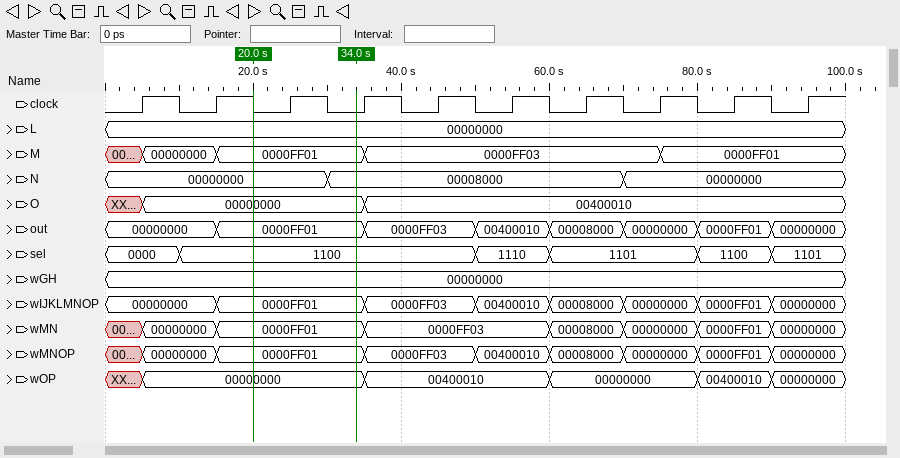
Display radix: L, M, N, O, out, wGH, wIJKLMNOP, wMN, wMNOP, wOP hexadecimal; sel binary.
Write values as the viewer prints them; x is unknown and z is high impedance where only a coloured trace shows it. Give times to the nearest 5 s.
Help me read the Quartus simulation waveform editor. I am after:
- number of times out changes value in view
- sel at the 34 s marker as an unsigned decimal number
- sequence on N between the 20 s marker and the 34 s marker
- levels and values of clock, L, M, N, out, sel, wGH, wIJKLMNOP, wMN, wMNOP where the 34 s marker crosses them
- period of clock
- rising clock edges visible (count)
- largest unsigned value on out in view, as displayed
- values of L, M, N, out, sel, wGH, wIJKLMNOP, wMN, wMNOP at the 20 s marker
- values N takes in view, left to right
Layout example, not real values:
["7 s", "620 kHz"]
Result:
["7", "12", "00000000, 00008000", "clock=0, L=00000000, M=0000FF01, N=00008000, out=0000FF01, sel=1100, wGH=00000000, wIJKLMNOP=0000FF01, wMN=0000FF01, wMNOP=0000FF01", "10 s", "10", "00400010", "L=00000000, M=0000FF01, N=00000000, out=0000FF01, sel=1100, wGH=00000000, wIJKLMNOP=0000FF01, wMN=0000FF01, wMNOP=0000FF01", "00000000, 00008000, 00000000"]
